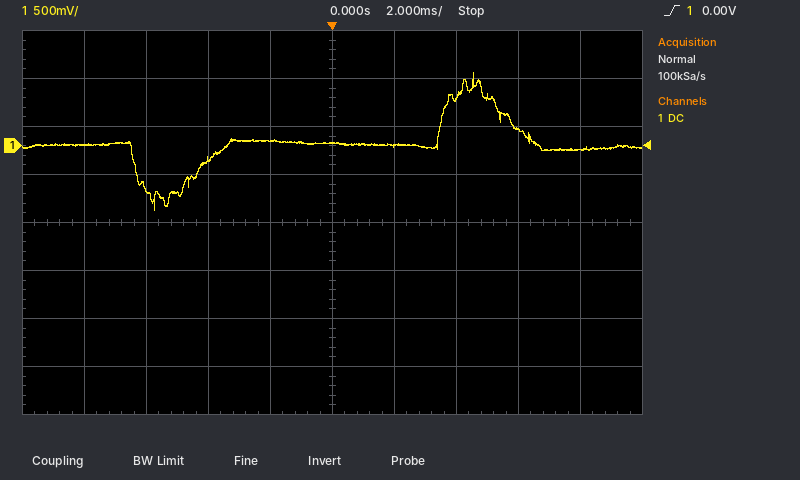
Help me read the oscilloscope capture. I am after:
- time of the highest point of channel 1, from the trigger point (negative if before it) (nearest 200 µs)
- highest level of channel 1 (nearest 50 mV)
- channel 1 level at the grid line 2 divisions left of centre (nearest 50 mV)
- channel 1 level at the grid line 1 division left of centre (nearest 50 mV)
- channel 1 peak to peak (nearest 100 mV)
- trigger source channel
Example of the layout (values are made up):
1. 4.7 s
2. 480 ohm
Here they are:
1. +4.6 ms
2. 750 mV
3. -150 mV
4. 50 mV
5. 1.40 V
6. channel 1
